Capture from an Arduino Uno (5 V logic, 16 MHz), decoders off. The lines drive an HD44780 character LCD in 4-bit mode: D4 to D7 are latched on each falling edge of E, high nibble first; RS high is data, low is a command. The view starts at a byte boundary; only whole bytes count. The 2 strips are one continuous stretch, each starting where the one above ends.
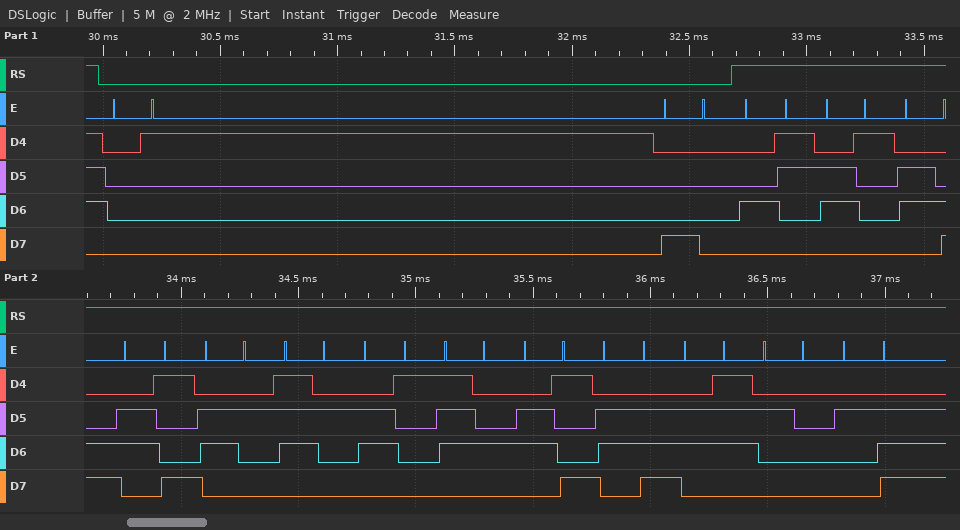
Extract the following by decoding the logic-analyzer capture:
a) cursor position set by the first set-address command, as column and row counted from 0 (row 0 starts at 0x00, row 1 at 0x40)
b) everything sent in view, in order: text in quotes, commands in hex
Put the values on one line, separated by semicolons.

column 0, row 0; 0x01 0x80 "Calibrating ."
